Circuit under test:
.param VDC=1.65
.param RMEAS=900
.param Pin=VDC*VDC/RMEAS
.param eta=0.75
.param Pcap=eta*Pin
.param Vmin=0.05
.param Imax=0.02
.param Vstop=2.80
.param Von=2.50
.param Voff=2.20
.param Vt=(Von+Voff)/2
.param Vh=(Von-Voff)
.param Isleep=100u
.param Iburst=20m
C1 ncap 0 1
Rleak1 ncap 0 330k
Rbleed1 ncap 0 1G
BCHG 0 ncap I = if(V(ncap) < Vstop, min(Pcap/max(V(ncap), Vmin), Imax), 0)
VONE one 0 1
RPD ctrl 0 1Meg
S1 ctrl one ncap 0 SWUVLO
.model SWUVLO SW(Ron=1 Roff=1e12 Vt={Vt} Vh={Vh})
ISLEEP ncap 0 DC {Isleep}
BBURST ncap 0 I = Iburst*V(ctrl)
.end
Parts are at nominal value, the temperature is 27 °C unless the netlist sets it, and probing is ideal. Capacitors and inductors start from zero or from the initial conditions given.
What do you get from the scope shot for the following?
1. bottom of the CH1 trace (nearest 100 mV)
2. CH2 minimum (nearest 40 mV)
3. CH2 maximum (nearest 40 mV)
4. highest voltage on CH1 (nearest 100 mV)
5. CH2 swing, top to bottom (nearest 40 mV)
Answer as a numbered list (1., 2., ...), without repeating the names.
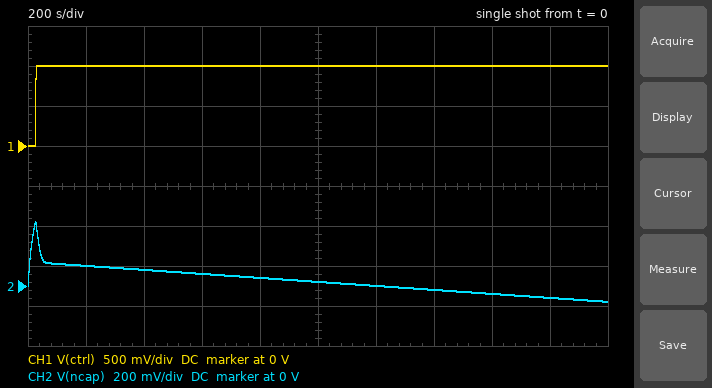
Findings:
1. 0 V
2. -80 mV
3. 320 mV
4. 1.0 V
5. 400 mV
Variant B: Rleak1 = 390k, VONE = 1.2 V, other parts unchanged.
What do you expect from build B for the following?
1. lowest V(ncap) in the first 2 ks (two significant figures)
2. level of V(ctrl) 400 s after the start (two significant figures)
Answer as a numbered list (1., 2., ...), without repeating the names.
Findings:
1. -270 mV
2. 1.2 V
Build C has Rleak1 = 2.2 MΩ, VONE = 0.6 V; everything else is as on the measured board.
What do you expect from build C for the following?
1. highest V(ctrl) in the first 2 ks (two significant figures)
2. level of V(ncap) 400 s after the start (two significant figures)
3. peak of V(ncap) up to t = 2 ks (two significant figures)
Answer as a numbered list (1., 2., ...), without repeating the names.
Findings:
1. 600 mV
2. 190 mV
3. 320 mV
